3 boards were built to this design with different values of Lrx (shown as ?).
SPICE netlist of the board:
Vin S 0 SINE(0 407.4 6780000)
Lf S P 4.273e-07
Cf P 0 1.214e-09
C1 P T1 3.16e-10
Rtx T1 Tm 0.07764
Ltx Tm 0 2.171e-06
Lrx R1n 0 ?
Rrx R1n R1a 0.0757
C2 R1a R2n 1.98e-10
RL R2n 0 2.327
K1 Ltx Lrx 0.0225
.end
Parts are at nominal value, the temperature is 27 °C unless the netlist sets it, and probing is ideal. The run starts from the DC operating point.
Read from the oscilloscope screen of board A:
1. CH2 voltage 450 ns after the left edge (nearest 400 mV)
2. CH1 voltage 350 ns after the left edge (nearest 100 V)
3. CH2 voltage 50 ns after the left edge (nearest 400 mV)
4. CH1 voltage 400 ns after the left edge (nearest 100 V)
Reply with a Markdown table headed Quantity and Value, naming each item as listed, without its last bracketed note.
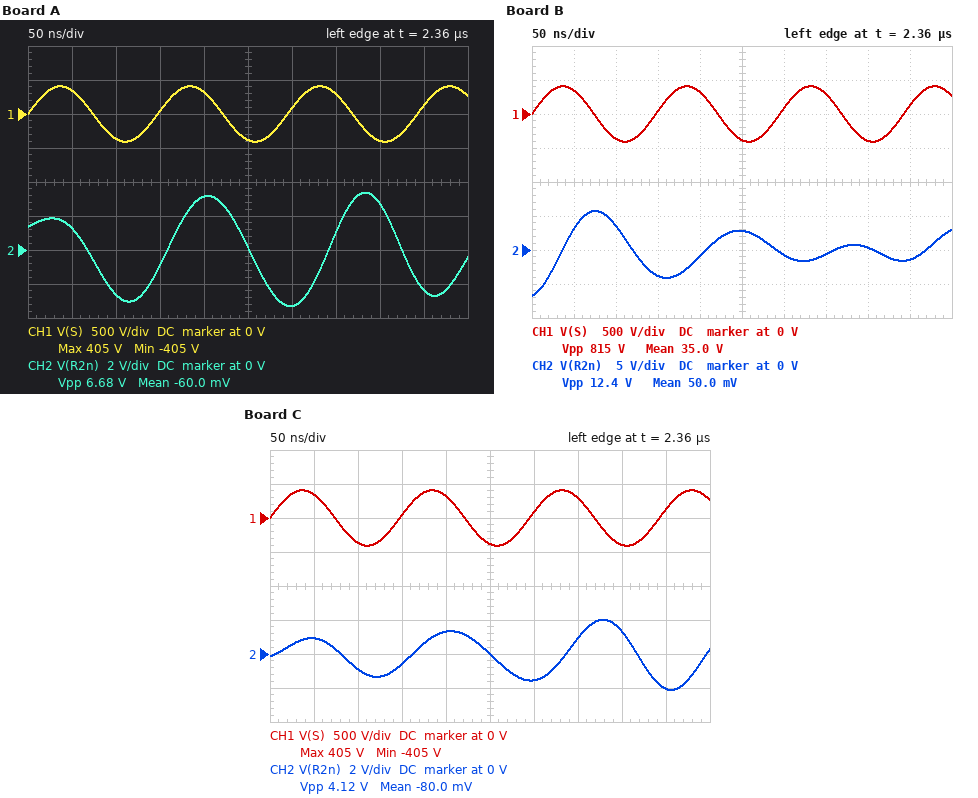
| Quantity | Value |
|---|---|
| CH2 voltage 450 ns after the left edge | -2.4 V |
| CH1 voltage 350 ns after the left edge | 300 V |
| CH2 voltage 50 ns after the left edge | 1.2 V |
| CH1 voltage 400 ns after the left edge | -400 V |
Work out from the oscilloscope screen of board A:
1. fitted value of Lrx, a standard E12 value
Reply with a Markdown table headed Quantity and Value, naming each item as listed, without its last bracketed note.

| Quantity | Value |
|---|---|
| fitted value of Lrx, a standard E12 value | 5.6 µH |
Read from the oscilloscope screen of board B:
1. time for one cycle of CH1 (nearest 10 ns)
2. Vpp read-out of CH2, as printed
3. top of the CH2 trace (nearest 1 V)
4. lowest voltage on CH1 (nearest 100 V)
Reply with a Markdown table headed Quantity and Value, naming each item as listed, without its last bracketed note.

| Quantity | Value |
|---|---|
| time for one cycle of CH1 | 150 ns |
| Vpp read-out of CH2, as printed | 12.4 V |
| top of the CH2 trace | 6 V |
| lowest voltage on CH1 | -400 V |
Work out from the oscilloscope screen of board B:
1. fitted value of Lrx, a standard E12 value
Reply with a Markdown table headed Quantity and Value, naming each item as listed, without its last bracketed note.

| Quantity | Value |
|---|---|
| fitted value of Lrx, a standard E12 value | 3.9 µH |
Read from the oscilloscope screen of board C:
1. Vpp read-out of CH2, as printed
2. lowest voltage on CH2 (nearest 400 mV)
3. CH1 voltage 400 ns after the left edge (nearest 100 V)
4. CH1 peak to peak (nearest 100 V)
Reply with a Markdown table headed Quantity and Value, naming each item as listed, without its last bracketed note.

| Quantity | Value |
|---|---|
| Vpp read-out of CH2, as printed | 4.12 V |
| lowest voltage on CH2 | -2.0 V |
| CH1 voltage 400 ns after the left edge | -400 V |
| CH1 peak to peak | 800 V |
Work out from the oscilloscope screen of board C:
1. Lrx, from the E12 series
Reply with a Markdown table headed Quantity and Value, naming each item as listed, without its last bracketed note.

| Quantity | Value |
|---|---|
| Lrx, from the E12 series | 6.8 µH |
